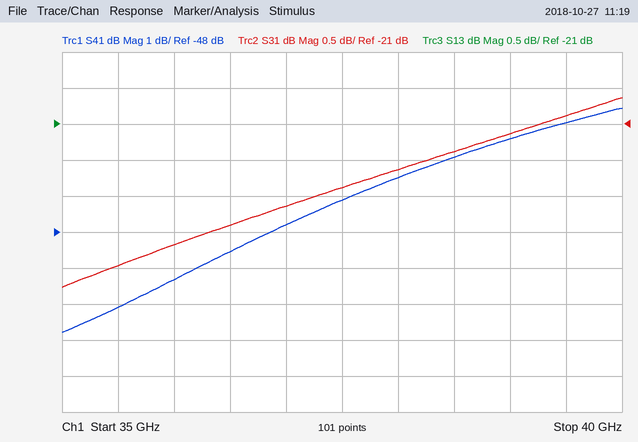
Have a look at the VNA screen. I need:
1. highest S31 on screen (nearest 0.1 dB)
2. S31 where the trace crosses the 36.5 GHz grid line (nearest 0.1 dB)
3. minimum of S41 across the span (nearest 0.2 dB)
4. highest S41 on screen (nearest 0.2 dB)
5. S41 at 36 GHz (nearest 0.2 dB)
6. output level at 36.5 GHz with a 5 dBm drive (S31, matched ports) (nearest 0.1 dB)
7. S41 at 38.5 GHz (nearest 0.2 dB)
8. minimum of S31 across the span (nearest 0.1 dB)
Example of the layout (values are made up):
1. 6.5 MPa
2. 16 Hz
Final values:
1. -20.6 dB
2. -22.4 dB
3. -50.8 dB
4. -44.6 dB
5. -49.4 dB
6. -17.4 dBm
7. -46.0 dB
8. -23.3 dB
